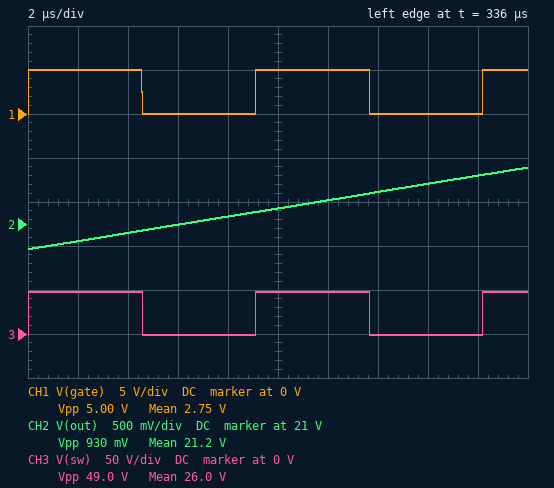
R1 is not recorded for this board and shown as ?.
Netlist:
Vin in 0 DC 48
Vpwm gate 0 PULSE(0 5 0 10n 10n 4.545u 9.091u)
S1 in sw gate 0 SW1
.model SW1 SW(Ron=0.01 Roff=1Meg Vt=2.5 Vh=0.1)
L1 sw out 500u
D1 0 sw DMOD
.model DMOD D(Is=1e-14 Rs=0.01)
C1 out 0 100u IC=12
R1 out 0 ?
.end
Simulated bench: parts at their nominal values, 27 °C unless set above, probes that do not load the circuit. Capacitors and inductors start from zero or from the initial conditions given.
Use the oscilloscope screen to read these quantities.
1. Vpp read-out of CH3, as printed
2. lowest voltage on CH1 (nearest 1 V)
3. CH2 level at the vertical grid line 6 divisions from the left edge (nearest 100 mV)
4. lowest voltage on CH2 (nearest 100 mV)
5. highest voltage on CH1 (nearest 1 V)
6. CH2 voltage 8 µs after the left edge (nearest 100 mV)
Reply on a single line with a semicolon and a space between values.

49.0 V; 0 V; 21.3 V; 20.7 V; 5 V; 21.1 V
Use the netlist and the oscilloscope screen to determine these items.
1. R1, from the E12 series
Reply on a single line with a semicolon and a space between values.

15 Ω
